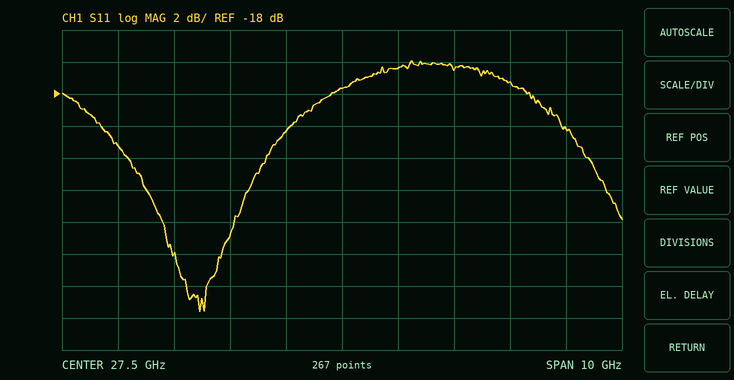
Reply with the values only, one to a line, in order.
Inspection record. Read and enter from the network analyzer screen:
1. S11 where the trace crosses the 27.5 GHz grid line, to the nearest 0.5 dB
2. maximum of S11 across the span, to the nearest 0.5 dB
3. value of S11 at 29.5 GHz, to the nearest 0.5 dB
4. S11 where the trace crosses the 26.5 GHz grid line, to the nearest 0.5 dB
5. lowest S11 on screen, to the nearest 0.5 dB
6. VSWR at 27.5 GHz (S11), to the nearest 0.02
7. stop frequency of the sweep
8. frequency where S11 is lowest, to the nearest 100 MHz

-17.5 dB
-16.0 dB
-16.5 dB
-20.5 dB
-31.5 dB
1.30
32.5 GHz
25.0 GHz
